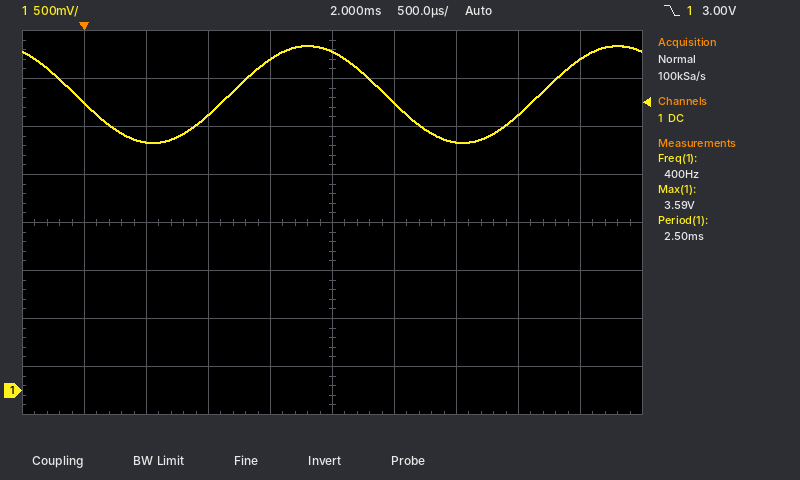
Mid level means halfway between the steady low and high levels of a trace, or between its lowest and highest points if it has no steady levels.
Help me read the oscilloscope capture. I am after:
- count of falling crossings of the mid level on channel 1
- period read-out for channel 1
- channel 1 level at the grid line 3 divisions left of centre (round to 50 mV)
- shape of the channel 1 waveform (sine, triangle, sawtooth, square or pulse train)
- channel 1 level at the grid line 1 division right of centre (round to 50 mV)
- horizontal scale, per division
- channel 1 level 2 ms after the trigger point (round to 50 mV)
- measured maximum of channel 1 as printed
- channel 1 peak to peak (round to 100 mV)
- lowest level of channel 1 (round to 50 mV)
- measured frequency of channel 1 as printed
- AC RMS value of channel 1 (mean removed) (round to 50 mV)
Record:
2
2.50 ms
2.60 V
sine
3.00 V
500 µs
3.55 V
3.59 V
1.00 V
2.60 V
400 Hz
350 mV
